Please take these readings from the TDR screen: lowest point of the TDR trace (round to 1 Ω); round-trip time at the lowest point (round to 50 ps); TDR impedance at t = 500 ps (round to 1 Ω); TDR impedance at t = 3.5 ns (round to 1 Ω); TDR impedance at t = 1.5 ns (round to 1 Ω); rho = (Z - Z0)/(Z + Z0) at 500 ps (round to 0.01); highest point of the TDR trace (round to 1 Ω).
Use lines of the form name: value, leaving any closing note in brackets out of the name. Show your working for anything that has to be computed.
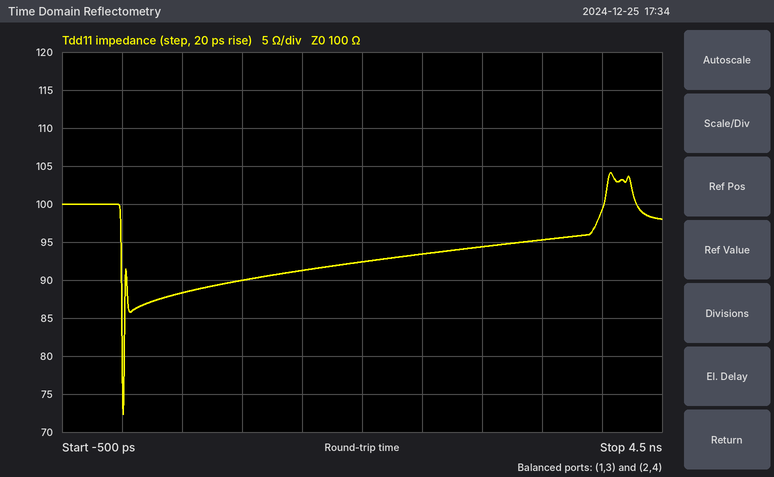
lowest point of the TDR trace: 72 Ω
round-trip time at the lowest point: 0 ps
TDR impedance at t = 500 ps: 88 Ω
TDR impedance at t = 3.5 ns: 95 Ω
TDR impedance at t = 1.5 ns: 91 Ω
rho = (Z - Z0)/(Z + Z0) at 500 ps: (88 − 100)/(88 + 100) ≈ -0.06
highest point of the TDR trace: 104 Ω
